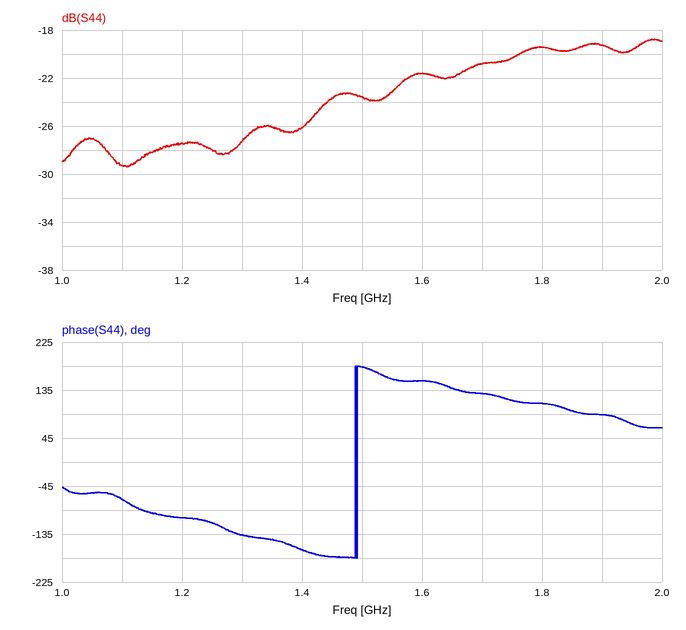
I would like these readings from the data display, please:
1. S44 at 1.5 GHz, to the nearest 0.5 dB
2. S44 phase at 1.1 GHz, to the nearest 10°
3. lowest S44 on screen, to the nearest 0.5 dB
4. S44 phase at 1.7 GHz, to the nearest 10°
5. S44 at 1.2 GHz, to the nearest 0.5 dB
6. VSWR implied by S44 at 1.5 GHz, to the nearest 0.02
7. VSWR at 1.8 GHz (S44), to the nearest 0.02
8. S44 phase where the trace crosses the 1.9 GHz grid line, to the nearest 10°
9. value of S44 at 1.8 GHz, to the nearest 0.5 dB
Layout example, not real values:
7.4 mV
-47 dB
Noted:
-23.5 dB
-70°
-29.5 dB
130°
-27.5 dB
1.14
1.24
90°
-19.5 dB
